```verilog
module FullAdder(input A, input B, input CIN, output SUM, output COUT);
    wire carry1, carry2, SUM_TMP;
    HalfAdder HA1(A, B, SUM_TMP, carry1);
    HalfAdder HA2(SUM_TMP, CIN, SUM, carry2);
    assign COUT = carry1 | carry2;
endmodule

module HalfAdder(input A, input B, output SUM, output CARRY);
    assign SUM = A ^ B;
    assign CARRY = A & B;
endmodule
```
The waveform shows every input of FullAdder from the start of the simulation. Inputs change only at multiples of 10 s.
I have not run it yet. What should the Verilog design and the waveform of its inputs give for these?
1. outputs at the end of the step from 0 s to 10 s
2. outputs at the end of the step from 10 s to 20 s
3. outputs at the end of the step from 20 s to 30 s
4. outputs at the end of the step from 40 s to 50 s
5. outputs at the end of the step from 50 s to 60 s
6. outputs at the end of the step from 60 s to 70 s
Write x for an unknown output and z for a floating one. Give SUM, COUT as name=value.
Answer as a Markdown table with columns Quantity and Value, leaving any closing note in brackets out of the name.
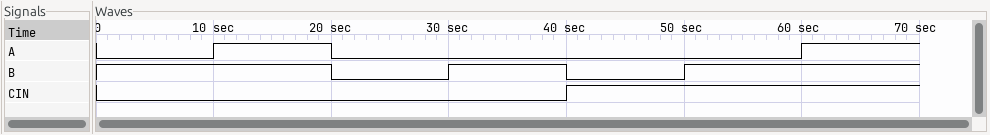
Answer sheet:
| Quantity | Value |
|---|---|
| outputs at the end of the step from 0 s to 10 s | SUM=1, COUT=0 |
| outputs at the end of the step from 10 s to 20 s | SUM=0, COUT=1 |
| outputs at the end of the step from 20 s to 30 s | SUM=0, COUT=0 |
| outputs at the end of the step from 40 s to 50 s | SUM=1, COUT=0 |
| outputs at the end of the step from 50 s to 60 s | SUM=0, COUT=1 |
| outputs at the end of the step from 60 s to 70 s | SUM=1, COUT=1 |
